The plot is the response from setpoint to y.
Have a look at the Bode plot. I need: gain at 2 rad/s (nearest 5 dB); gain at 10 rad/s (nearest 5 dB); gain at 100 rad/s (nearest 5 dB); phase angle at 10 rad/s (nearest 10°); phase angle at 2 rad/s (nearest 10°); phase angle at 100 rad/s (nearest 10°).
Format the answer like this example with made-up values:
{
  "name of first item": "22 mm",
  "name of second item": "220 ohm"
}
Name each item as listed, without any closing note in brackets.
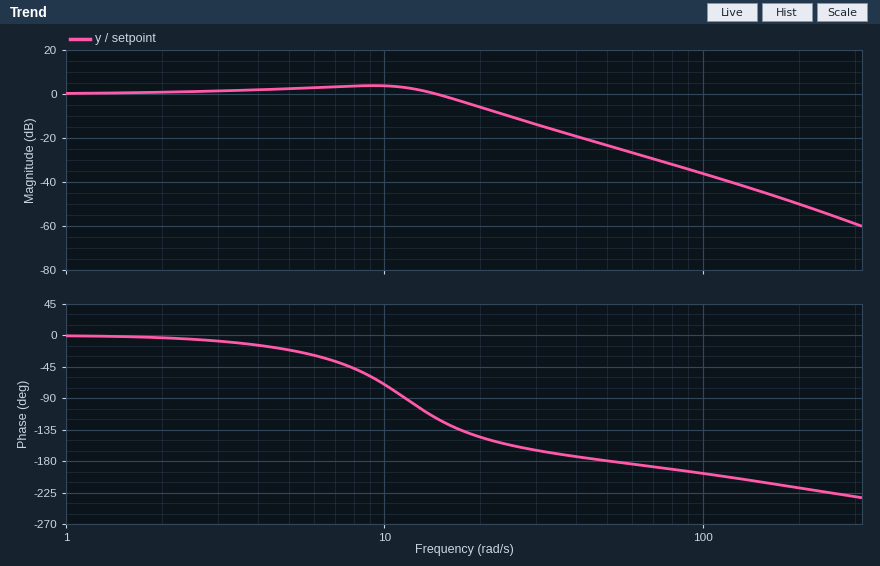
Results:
{
  "gain at 2 rad/s": "0 dB",
  "gain at 10 rad/s": "5 dB",
  "gain at 100 rad/s": "-35 dB",
  "phase angle at 10 rad/s": "-70°",
  "phase angle at 2 rad/s": "0°",
  "phase angle at 100 rad/s": "-200°"
}
